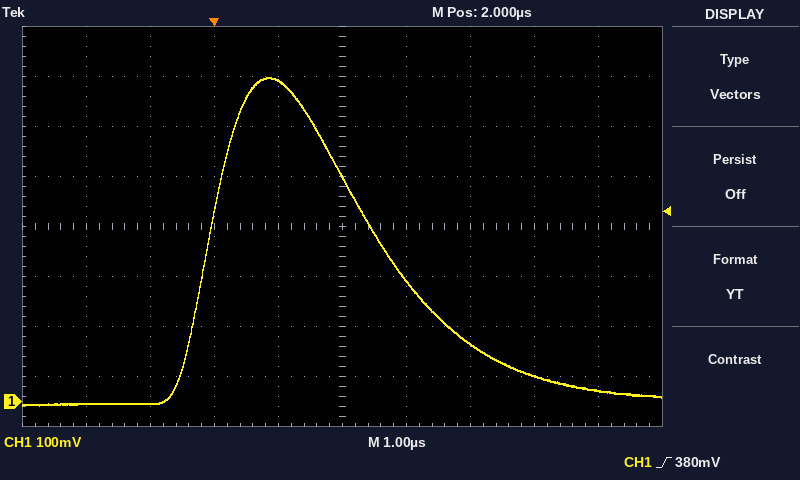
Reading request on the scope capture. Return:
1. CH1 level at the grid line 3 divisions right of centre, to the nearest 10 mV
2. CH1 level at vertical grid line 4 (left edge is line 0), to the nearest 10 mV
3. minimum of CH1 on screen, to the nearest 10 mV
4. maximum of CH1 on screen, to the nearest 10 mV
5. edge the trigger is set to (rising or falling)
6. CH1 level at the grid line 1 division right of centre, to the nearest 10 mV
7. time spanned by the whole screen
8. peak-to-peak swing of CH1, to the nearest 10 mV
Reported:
50 mV
640 mV
-10 mV
650 mV
rising
240 mV
10 µs
660 mV
